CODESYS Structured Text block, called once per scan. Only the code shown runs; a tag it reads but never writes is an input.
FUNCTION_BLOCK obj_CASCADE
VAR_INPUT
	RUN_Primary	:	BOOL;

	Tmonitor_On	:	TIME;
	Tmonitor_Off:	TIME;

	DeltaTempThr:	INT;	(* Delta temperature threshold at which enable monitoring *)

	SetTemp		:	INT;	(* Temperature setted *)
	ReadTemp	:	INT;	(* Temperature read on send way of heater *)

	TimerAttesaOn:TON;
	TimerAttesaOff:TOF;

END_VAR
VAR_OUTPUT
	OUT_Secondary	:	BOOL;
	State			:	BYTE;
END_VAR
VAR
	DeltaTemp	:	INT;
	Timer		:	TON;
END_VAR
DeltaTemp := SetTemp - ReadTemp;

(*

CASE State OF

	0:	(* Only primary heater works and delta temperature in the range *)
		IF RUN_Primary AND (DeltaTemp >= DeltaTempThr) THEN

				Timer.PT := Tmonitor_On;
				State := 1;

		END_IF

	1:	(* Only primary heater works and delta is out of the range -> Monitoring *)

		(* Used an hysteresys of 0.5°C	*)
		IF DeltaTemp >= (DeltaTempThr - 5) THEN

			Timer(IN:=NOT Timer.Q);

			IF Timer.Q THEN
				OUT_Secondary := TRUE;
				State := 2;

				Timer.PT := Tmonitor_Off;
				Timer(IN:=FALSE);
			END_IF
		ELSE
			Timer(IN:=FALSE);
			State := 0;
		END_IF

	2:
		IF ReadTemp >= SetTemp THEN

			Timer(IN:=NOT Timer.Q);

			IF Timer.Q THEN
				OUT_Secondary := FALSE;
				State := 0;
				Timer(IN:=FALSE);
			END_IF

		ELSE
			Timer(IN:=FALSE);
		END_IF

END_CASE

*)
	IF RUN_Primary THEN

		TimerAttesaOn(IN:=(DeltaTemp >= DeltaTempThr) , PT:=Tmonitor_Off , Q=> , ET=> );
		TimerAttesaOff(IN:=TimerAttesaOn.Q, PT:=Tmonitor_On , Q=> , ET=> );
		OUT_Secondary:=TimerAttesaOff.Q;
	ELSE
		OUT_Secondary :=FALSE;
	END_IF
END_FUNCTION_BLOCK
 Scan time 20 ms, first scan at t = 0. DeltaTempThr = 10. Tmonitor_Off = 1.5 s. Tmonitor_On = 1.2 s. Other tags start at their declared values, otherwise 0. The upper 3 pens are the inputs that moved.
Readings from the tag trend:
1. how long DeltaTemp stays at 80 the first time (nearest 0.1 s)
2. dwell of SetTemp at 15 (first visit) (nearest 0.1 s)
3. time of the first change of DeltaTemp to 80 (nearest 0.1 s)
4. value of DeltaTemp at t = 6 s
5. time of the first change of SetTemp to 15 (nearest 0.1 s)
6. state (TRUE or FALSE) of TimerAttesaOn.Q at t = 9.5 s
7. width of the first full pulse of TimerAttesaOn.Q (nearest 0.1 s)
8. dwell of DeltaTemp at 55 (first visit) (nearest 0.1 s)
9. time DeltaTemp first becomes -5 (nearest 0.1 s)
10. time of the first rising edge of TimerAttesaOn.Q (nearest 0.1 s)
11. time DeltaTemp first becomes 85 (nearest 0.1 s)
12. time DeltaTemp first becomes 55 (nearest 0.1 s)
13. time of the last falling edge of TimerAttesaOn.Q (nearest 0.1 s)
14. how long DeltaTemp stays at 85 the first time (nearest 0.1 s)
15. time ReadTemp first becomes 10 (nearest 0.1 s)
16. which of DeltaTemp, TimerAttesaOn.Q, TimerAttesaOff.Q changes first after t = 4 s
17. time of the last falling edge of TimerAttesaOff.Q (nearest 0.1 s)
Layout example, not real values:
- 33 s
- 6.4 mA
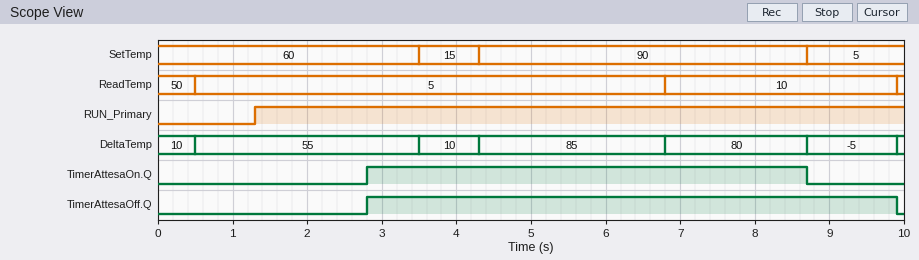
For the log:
- 1.9 s
- 0.8 s
- 6.8 s
- 85
- 3.5 s
- FALSE
- 5.9 s
- 3.0 s
- 8.7 s
- 2.8 s
- 4.3 s
- 0.5 s
- 8.7 s
- 2.5 s
- 6.8 s
- DeltaTemp
- 9.9 s
